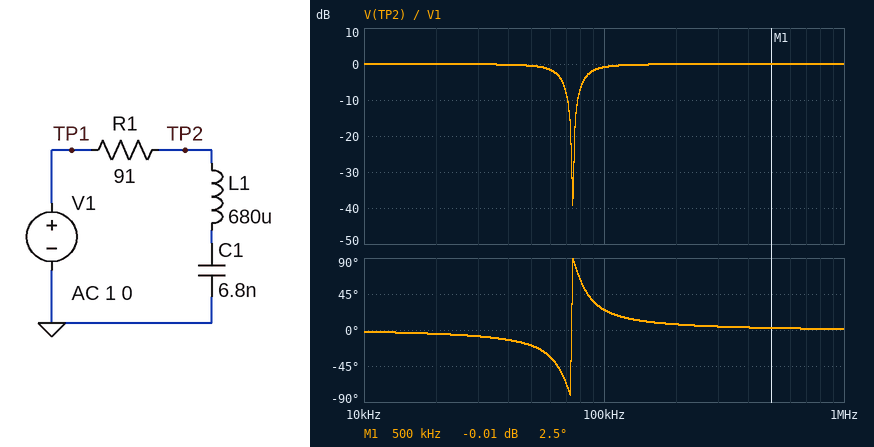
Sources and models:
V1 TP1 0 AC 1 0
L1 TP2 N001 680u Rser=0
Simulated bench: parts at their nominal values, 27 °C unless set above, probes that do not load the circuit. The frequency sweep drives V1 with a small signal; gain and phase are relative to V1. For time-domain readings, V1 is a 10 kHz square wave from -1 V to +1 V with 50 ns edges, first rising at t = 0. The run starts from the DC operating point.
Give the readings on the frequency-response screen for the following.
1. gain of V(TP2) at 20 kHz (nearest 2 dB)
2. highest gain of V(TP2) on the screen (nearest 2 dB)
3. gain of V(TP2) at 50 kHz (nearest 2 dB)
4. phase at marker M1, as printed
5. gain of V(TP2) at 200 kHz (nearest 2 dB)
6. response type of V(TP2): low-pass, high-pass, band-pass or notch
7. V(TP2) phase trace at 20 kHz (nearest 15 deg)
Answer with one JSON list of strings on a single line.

["0 dB", "0 dB", "0 dB", "2.5 deg", "0 dB", "notch", "0 deg"]
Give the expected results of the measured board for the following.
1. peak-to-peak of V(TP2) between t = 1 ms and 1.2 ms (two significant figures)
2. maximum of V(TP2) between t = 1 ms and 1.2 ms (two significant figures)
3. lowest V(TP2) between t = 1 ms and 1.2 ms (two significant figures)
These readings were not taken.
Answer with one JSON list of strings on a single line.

["2.6 V", "1.3 V", "-1.3 V"]
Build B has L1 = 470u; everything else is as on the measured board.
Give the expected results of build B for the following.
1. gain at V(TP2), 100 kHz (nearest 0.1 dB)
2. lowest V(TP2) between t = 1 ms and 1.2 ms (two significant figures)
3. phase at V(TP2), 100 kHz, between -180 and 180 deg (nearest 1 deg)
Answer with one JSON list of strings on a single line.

["-5.1 dB", "-1.3 V", "56 deg"]
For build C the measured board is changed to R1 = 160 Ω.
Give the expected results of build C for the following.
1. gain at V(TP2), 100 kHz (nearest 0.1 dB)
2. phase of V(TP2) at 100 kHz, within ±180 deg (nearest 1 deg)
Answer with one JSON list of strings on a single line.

["-2.3 dB", "40 deg"]
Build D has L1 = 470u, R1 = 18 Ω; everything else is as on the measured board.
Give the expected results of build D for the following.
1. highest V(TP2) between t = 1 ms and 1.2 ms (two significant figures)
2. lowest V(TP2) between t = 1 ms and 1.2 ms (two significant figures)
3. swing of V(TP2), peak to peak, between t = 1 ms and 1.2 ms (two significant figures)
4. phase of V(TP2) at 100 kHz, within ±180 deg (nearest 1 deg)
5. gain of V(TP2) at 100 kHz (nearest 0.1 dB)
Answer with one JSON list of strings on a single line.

["1.2 V", "-1.2 V", "2.4 V", "16 deg", "-0.4 dB"]
